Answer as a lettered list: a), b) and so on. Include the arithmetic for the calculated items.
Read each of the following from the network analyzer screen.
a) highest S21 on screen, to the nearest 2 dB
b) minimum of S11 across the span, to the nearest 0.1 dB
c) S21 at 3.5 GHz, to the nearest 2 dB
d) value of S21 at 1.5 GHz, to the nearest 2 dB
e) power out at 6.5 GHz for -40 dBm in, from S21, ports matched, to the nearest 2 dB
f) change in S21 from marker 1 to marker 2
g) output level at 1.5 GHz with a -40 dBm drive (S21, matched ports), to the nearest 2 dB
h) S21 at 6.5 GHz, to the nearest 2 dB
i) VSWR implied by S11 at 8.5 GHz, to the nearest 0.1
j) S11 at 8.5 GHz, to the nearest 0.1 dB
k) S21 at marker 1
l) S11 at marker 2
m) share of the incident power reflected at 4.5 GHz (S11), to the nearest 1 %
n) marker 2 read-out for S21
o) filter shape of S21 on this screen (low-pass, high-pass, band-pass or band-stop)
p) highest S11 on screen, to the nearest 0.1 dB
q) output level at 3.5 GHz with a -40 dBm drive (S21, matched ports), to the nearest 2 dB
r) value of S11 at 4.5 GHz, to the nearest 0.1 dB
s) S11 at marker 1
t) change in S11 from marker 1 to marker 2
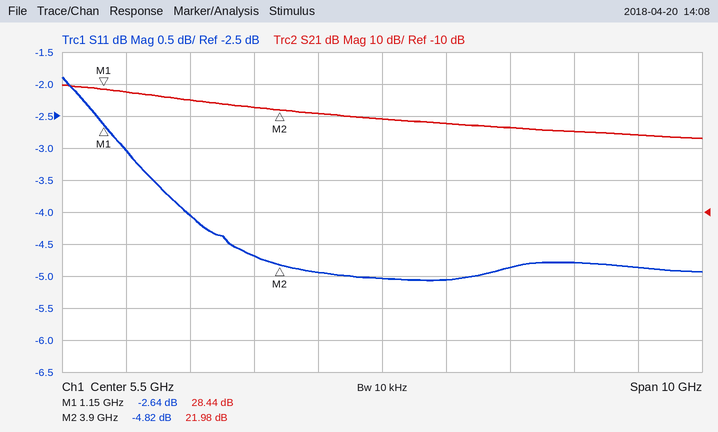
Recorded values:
a) 30 dB
b) -5.1 dB
c) 22 dB
d) 28 dB
e) -40 dBm + (18 dB) = -22 dBm
f) 21.98 − (28.44) = -6.46 dB
g) -40 dBm + (28 dB) = -12 dBm
h) 18 dB
i) |Γ| = 10^(-4.8/20) = 0.5754; VSWR = (1 + 0.5754)/(1 − 0.5754) ≈ 3.7
j) -4.8 dB
k) 28.44 dB
l) -4.82 dB
m) 10^(-4.9/10) ≈ 32 %
n) 21.98 dB
o) low-pass
p) -1.9 dB
q) -40 dBm + (22 dB) = -18 dBm
r) -4.9 dB
s) -2.64 dB
t) -4.82 − (-2.64) = -2.18 dB
